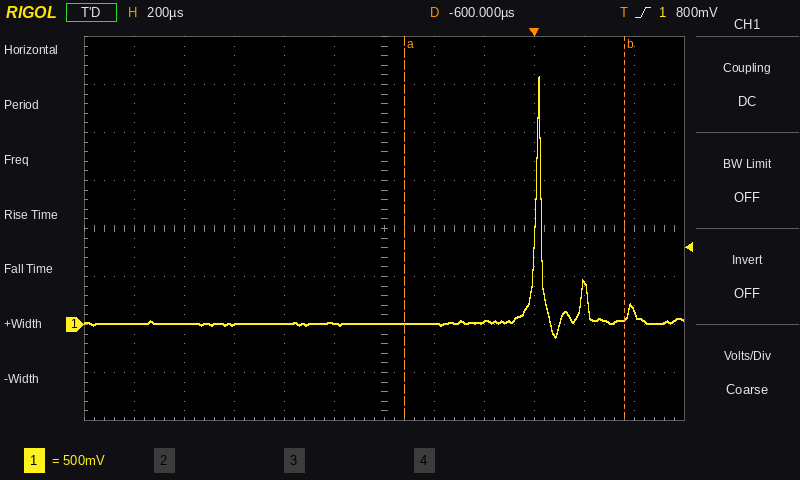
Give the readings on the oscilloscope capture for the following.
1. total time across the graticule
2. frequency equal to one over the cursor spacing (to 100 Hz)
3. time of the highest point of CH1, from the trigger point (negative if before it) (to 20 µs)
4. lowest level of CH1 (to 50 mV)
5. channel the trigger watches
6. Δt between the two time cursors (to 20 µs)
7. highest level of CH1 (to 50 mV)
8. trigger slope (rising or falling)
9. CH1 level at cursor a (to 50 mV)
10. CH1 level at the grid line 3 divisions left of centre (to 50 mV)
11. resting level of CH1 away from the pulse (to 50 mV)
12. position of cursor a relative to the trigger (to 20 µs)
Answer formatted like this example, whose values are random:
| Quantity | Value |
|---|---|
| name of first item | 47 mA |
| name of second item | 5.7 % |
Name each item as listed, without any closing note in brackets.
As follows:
| Quantity | Value |
|---|---|
| total time across the graticule | 2.4 ms |
| frequency equal to one over the cursor spacing | 1.1 kHz |
| time of the highest point of CH1, from the trigger point (negative if before it) | +20 µs |
| lowest level of CH1 | -150 mV |
| channel the trigger watches | CH1 |
| Δt between the two time cursors | 880 µs |
| highest level of CH1 | 2.60 V |
| trigger slope | rising |
| CH1 level at cursor a | 0 mV |
| CH1 level at the grid line 3 divisions left of centre | 0 mV |
| resting level of CH1 away from the pulse | 0 mV |
| position of cursor a relative to the trigger | -520 µs |
